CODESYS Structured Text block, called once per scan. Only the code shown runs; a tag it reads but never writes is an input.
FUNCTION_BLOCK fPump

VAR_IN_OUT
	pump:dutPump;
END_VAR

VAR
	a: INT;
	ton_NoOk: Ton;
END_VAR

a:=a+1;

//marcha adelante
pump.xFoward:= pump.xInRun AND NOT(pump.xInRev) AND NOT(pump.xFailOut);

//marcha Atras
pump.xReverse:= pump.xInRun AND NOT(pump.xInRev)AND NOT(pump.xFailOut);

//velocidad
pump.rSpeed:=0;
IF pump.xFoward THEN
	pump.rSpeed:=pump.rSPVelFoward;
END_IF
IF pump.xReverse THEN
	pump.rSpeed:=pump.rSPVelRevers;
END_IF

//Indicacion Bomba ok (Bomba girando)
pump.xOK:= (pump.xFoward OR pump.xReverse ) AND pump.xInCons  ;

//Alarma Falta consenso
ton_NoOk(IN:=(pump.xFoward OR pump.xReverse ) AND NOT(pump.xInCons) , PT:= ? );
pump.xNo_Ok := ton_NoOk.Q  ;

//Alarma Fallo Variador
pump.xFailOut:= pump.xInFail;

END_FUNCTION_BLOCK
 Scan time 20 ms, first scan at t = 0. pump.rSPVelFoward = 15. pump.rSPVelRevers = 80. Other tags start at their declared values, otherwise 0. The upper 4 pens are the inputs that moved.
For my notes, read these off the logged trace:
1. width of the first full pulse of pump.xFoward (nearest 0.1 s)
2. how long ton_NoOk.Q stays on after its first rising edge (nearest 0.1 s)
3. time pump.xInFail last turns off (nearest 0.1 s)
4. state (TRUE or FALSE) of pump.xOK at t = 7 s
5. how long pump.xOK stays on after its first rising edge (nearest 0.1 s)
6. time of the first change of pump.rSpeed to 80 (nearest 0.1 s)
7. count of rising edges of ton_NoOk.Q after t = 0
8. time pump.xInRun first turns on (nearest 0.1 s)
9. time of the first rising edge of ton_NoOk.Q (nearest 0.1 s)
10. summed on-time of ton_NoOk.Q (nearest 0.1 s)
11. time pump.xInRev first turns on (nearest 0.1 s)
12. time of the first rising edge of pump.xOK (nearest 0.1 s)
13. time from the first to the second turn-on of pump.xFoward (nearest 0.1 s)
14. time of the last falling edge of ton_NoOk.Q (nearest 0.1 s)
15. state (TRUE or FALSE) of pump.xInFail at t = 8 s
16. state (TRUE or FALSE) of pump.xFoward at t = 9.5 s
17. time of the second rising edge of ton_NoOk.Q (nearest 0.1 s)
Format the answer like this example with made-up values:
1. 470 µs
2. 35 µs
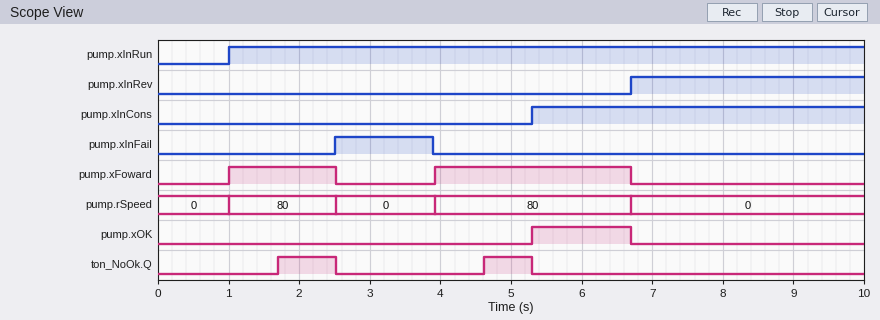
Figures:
1. 1.5 s
2. 0.8 s
3. 3.9 s
4. FALSE
5. 1.4 s
6. 1.0 s
7. 2
8. 1.0 s
9. 1.7 s
10. 1.5 s
11. 6.7 s
12. 5.3 s
13. 2.9 s
14. 5.3 s
15. FALSE
16. FALSE
17. 4.6 s
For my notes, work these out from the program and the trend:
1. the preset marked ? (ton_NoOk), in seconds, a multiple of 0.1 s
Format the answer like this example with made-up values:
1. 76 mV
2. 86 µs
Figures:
1. 0.7 s
